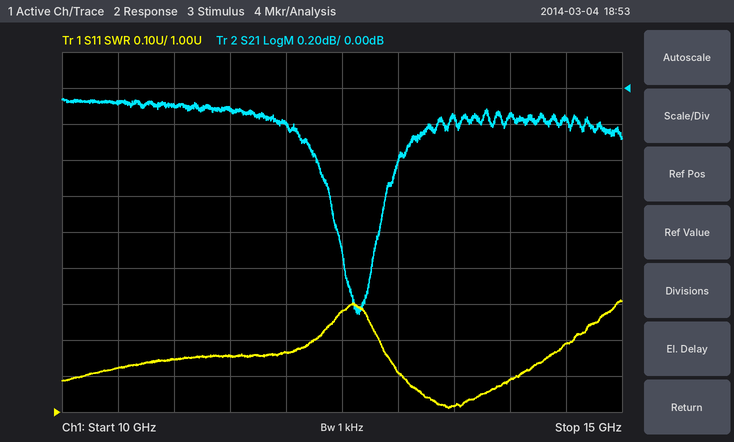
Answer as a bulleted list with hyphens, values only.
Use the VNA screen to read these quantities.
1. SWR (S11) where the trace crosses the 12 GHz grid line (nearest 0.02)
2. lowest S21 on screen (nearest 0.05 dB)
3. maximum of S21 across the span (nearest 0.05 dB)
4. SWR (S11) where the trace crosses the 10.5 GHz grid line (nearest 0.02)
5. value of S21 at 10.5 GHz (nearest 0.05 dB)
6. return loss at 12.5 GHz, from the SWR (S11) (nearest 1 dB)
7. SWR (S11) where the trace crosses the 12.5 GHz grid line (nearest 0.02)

- 1.16
- -1.25 dB
- -0.05 dB
- 1.12
- -0.10 dB
- 18 dB
- 1.28
